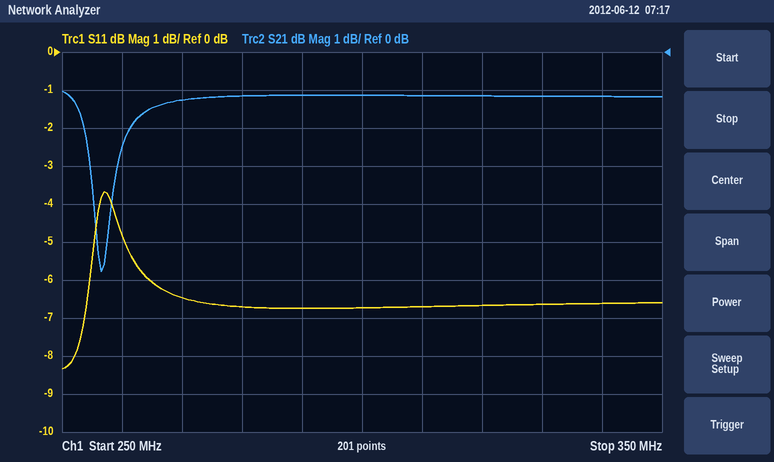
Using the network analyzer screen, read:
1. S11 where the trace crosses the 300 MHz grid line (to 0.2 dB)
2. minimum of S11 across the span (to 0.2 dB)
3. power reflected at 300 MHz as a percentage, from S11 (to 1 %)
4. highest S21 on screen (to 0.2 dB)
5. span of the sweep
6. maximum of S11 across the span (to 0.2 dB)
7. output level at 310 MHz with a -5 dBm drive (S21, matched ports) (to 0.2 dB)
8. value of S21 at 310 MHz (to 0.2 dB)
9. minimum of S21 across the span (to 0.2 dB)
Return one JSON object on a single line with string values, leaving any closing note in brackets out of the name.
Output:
{"S11 where the trace crosses the 300 MHz grid line": "-6.8 dB", "minimum of S11 across the span": "-8.4 dB", "power reflected at 300 MHz as a percentage, from S11": "21 %", "highest S21 on screen": "-1.0 dB", "span of the sweep": "100 MHz", "maximum of S11 across the span": "-3.6 dB", "output level at 310 MHz with a -5 dBm drive (S21, matched ports)": "-6.2 dBm", "value of S21 at 310 MHz": "-1.2 dB", "minimum of S21 across the span": "-5.8 dB"}
